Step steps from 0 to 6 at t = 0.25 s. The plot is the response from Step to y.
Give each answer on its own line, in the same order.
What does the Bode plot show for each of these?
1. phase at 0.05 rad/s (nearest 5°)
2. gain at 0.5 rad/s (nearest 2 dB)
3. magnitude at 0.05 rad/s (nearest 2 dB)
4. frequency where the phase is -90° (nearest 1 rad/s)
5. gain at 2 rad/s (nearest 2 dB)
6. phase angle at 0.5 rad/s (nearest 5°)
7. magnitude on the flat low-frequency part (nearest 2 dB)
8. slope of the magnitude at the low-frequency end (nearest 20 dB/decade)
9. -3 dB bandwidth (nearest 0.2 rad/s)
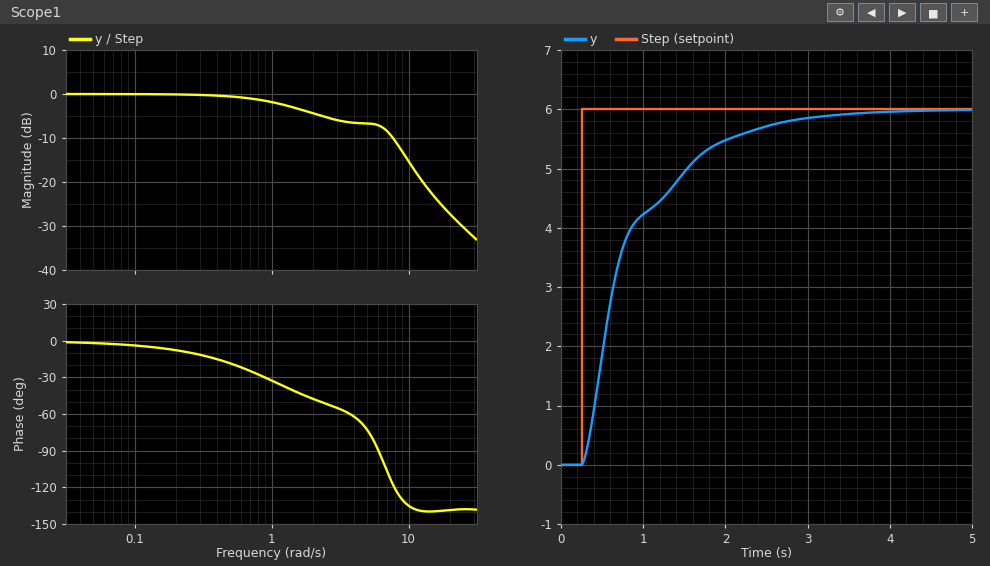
0°
0 dB
0 dB
6 rad/s
-4 dB
-20°
0 dB
0 dB/decade
1.4 rad/s
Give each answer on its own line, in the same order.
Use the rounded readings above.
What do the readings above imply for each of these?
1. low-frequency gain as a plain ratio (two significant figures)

1.0
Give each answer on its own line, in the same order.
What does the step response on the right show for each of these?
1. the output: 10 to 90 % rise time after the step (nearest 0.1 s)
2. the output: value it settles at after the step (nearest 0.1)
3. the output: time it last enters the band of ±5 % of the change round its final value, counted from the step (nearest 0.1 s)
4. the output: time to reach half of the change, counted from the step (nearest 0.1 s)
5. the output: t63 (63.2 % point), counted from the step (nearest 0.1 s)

1.5 s
6.0
2.2 s
0.4 s
0.5 s
